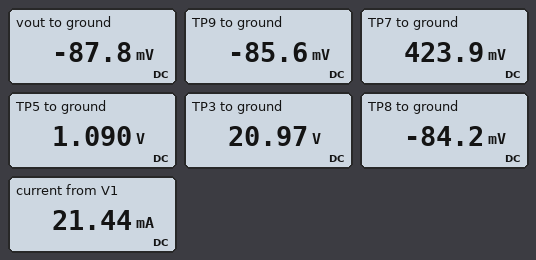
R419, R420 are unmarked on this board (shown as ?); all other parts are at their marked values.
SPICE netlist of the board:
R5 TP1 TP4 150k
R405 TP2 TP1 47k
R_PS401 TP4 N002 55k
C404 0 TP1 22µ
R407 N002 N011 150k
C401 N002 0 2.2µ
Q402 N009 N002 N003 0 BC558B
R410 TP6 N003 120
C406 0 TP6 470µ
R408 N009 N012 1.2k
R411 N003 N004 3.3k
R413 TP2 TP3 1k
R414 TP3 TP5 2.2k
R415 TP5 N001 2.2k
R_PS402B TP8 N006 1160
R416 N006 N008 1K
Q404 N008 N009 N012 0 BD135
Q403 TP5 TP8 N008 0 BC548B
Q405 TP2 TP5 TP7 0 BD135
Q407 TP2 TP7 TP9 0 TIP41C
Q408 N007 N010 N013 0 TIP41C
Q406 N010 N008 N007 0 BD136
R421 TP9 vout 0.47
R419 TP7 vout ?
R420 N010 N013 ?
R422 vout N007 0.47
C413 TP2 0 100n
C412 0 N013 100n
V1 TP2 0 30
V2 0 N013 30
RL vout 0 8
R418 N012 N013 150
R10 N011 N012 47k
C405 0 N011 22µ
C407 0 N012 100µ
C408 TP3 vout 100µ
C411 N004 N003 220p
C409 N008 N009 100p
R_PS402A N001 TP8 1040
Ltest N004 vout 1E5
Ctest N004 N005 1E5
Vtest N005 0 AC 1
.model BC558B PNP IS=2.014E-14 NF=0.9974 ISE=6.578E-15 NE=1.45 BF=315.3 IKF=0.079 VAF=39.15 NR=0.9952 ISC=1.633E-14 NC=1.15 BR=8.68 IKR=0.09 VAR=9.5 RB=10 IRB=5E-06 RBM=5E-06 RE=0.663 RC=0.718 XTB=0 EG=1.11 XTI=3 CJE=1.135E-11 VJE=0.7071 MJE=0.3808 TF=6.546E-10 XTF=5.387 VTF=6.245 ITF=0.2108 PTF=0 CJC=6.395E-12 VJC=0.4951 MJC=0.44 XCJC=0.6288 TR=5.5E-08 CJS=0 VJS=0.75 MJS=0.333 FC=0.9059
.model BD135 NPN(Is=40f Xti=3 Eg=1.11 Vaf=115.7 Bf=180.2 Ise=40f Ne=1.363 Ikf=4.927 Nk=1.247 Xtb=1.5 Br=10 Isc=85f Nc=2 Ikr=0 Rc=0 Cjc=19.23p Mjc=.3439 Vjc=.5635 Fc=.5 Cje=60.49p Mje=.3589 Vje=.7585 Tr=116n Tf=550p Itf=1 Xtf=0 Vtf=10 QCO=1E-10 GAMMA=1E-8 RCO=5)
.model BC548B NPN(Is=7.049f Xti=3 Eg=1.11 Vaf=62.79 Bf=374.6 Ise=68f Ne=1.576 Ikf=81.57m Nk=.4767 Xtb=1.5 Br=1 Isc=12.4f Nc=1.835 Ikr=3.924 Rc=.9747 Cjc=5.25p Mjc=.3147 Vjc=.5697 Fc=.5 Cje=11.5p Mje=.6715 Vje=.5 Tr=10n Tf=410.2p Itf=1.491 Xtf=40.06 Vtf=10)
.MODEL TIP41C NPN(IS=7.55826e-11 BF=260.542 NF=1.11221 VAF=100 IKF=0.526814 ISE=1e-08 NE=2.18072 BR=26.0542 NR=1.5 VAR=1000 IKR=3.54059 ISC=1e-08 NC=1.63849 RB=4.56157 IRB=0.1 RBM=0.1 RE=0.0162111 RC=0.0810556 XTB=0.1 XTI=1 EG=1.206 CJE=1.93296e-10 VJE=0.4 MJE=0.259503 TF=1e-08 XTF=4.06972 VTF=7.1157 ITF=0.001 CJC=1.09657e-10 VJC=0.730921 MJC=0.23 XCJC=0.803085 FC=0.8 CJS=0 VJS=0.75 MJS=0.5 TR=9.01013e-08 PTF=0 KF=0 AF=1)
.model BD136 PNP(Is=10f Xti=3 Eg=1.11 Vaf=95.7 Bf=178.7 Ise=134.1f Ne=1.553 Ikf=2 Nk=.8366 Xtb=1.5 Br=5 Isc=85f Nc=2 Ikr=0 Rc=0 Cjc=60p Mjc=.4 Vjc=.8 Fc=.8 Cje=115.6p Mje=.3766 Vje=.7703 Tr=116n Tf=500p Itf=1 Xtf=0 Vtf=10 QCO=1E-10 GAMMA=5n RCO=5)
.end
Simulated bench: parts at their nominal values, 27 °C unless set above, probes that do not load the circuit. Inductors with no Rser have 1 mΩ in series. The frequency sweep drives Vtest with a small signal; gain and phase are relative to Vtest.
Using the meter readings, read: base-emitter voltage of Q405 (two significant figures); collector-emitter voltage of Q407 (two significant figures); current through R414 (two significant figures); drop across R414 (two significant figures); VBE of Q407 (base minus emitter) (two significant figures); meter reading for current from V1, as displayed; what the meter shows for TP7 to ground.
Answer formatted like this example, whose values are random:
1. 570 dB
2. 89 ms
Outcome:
1. 670 mV
2. 30 V
3. 9.0 mA
4. 20 V
5. 510 mV
6. 21.44 mA
7. 423.9 mV
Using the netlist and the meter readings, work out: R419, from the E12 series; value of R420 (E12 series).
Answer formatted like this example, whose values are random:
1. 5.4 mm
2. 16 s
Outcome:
1. 68 Ω
2. 56 Ω
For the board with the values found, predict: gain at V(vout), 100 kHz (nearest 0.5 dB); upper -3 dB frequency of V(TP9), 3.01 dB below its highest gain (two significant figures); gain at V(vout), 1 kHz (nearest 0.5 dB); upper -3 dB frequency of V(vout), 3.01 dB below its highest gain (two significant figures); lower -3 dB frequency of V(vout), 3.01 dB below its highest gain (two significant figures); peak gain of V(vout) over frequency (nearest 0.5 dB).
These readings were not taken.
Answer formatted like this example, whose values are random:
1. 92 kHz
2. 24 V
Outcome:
1. 10.5 dB
2. 1.4 kHz
3. 45.0 dB
4. 1.4 kHz
5. 4.9 Hz
6. 47.0 dB
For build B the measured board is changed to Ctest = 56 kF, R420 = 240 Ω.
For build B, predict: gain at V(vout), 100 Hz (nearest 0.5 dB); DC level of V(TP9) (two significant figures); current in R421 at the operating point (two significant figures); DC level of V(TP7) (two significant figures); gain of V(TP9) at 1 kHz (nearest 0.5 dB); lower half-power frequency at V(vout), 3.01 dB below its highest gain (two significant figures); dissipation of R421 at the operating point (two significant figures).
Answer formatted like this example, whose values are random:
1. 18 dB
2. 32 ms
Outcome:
1. 48.5 dB
2. -88 mV
3. 11 mA
4. 450 mV
5. 46.5 dB
6. 7.5 Hz
7. 60 µW
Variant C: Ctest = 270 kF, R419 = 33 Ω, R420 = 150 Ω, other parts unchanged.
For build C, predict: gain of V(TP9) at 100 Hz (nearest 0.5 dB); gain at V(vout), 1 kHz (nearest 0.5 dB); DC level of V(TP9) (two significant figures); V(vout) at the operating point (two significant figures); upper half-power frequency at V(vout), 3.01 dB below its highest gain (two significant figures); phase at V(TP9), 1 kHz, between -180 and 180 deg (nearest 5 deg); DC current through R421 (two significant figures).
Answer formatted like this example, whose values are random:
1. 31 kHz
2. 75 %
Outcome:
1. 48.0 dB
2. 46.0 dB
3. -94 mV
4. -96 mV
5. 1.2 kHz
6. 140 deg
7. 4.7 mA
